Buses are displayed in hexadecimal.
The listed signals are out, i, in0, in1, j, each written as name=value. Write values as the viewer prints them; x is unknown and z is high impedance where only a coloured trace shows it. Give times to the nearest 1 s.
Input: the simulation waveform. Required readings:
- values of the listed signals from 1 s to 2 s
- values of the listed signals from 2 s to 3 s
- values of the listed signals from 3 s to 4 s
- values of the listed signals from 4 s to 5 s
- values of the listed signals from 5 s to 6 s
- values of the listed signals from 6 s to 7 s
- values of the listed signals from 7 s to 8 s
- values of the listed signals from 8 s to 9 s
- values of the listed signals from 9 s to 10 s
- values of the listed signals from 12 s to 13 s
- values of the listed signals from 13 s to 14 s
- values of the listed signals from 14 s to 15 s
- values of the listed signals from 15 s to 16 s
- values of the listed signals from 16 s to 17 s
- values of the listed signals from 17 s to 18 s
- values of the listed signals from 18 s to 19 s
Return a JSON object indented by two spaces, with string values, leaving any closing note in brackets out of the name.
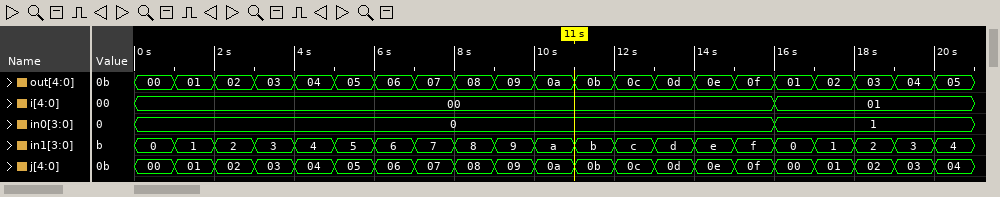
{
  "values of the listed signals from 1 s to 2 s": "out=01, i=00, in0=0, in1=1, j=01",
  "values of the listed signals from 2 s to 3 s": "out=02, i=00, in0=0, in1=2, j=02",
  "values of the listed signals from 3 s to 4 s": "out=03, i=00, in0=0, in1=3, j=03",
  "values of the listed signals from 4 s to 5 s": "out=04, i=00, in0=0, in1=4, j=04",
  "values of the listed signals from 5 s to 6 s": "out=05, i=00, in0=0, in1=5, j=05",
  "values of the listed signals from 6 s to 7 s": "out=06, i=00, in0=0, in1=6, j=06",
  "values of the listed signals from 7 s to 8 s": "out=07, i=00, in0=0, in1=7, j=07",
  "values of the listed signals from 8 s to 9 s": "out=08, i=00, in0=0, in1=8, j=08",
  "values of the listed signals from 9 s to 10 s": "out=09, i=00, in0=0, in1=9, j=09",
  "values of the listed signals from 12 s to 13 s": "out=0c, i=00, in0=0, in1=c, j=0c",
  "values of the listed signals from 13 s to 14 s": "out=0d, i=00, in0=0, in1=d, j=0d",
  "values of the listed signals from 14 s to 15 s": "out=0e, i=00, in0=0, in1=e, j=0e",
  "values of the listed signals from 15 s to 16 s": "out=0f, i=00, in0=0, in1=f, j=0f",
  "values of the listed signals from 16 s to 17 s": "out=01, i=01, in0=1, in1=0, j=00",
  "values of the listed signals from 17 s to 18 s": "out=02, i=01, in0=1, in1=1, j=01",
  "values of the listed signals from 18 s to 19 s": "out=03, i=01, in0=1, in1=2, j=02"
}
